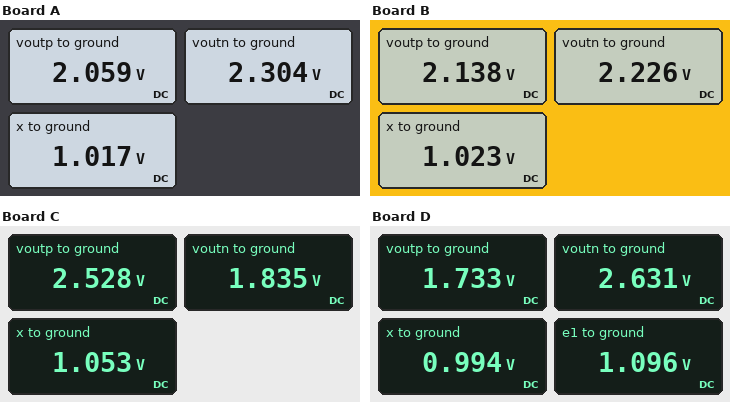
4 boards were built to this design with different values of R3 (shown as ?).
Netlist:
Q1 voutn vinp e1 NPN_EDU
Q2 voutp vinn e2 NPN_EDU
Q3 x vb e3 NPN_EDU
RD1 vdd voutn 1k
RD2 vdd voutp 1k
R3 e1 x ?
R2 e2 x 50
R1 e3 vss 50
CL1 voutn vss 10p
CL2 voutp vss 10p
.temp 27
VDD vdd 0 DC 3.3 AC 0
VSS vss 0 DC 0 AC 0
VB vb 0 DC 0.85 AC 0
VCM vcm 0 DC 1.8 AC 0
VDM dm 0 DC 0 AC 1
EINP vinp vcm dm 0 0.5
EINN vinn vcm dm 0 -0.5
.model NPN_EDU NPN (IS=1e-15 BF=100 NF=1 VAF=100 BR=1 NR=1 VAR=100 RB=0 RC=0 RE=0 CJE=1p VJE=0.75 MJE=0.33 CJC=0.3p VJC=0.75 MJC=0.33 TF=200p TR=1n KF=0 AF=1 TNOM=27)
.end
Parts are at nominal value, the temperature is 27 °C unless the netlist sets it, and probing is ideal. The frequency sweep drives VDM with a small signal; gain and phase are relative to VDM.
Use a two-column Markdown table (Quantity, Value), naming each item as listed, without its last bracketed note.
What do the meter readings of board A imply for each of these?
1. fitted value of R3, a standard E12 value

| Quantity | Value |
|---|---|
| fitted value of R3, a standard E12 value | 68 Ω |
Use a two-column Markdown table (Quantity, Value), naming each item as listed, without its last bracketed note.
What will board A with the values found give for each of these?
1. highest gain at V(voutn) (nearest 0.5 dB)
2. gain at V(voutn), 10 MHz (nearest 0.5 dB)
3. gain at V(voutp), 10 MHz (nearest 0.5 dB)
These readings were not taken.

| Quantity | Value |
|---|---|
| highest gain at V(voutn) | 15.5 dB |
| gain at V(voutn), 10 MHz | 14.0 dB |
| gain at V(voutp), 10 MHz | 14.0 dB |
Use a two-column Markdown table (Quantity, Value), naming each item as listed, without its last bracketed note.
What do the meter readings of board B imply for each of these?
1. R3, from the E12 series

| Quantity | Value |
|---|---|
| R3, from the E12 series | 56 Ω |
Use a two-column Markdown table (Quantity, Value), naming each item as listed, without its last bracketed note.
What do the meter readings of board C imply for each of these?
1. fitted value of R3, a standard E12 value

| Quantity | Value |
|---|---|
| fitted value of R3, a standard E12 value | 15 Ω |
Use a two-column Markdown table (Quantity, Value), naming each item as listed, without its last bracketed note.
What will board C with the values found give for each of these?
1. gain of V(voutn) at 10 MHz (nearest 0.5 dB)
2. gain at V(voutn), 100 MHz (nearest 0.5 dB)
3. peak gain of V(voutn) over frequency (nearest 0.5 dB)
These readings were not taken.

| Quantity | Value |
|---|---|
| gain of V(voutn) at 10 MHz | 17.0 dB |
| gain at V(voutn), 100 MHz | 2.5 dB |
| peak gain of V(voutn) over frequency | 18.5 dB |
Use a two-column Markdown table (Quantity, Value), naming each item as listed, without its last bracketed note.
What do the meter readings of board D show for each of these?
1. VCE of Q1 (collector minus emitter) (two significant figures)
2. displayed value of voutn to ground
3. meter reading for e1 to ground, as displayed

| Quantity | Value |
|---|---|
| VCE of Q1 (collector minus emitter) | 1.5 V |
| displayed value of voutn to ground | 2.631 V |
| meter reading for e1 to ground, as displayed | 1.096 V |
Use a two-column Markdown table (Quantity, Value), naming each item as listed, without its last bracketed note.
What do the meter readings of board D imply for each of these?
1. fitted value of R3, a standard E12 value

| Quantity | Value |
|---|---|
| fitted value of R3, a standard E12 value | 150 Ω |
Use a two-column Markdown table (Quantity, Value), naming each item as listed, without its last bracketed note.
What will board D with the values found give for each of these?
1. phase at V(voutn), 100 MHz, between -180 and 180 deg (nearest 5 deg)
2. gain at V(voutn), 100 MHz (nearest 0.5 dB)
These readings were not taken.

| Quantity | Value |
|---|---|
| phase at V(voutn), 100 MHz, between -180 and 180 deg | 90 deg |
| gain at V(voutn), 100 MHz | -4.5 dB |
